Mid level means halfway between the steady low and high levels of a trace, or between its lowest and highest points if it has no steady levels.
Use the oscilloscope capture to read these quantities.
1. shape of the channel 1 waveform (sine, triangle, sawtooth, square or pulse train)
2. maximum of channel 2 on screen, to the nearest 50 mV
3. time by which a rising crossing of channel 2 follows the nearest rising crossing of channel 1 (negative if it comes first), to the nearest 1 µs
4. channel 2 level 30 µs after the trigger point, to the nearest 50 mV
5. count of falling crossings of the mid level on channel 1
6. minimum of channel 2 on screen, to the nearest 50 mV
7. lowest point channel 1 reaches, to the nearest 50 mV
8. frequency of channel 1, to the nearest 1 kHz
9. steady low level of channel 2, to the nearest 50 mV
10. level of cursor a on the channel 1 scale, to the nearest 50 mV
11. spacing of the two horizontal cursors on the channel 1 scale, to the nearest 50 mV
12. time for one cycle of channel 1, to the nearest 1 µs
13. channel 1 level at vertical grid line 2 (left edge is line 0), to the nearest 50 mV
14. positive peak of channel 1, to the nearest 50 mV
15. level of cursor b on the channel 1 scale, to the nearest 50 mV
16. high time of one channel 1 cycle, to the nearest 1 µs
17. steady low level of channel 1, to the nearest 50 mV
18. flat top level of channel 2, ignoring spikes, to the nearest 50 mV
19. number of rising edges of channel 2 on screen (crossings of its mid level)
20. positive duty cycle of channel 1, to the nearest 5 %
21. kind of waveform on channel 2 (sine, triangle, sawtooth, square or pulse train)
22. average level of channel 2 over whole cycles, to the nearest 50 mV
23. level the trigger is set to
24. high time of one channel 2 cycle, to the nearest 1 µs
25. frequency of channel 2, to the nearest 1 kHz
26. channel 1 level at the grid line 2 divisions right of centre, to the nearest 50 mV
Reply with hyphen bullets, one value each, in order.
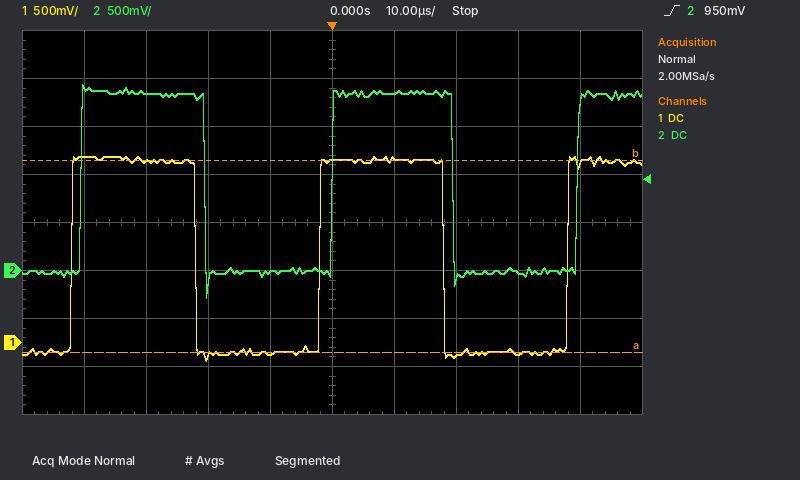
- square
- 1.95 V
- +2 µs
- 0 mV
- 2
- -300 mV
- -200 mV
- 25 kHz
- 0 mV
- -100 mV
- 2.00 V
- 40 µs
- 1.90 V
- 1.95 V
- 1.90 V
- 20 µs
- -100 mV
- 1.85 V
- 3
- 50 %
- square
- 900 mV
- 950 mV
- 20 µs
- 25 kHz
- -150 mV
